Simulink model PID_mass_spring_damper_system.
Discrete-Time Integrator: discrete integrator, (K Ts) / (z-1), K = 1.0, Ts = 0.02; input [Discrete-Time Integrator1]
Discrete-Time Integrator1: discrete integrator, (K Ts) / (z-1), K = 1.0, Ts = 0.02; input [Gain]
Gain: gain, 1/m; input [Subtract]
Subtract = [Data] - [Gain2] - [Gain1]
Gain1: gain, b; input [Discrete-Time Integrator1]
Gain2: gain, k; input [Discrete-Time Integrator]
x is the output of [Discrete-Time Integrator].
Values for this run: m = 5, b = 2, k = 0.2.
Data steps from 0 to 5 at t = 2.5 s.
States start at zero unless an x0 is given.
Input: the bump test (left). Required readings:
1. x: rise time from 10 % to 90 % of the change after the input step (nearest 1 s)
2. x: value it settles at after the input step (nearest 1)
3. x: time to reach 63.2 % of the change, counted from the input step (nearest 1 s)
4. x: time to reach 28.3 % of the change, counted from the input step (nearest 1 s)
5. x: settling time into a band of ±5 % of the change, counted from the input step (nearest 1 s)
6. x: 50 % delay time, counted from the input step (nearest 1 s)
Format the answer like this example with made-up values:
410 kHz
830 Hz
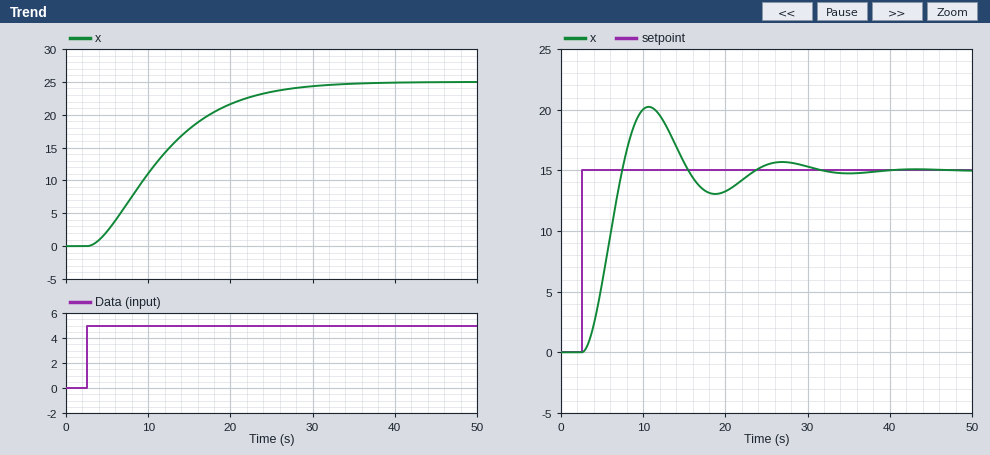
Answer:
17 s
25
11 s
5 s
24 s
8 s
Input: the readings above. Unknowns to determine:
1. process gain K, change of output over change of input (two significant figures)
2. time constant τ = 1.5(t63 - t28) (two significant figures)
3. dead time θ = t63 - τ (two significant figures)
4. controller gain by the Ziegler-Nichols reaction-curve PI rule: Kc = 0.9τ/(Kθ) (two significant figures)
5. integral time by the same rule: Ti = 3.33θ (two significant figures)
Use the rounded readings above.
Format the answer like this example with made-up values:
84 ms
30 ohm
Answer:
5.0
9.0 s
2.0 s
0.81
6.7 s
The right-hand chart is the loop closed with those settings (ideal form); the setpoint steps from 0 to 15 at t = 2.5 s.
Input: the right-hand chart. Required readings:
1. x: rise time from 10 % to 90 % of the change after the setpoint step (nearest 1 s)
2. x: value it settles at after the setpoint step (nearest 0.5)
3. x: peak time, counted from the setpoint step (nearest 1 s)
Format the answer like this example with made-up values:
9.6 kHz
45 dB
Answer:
3 s
15.0
8 s
